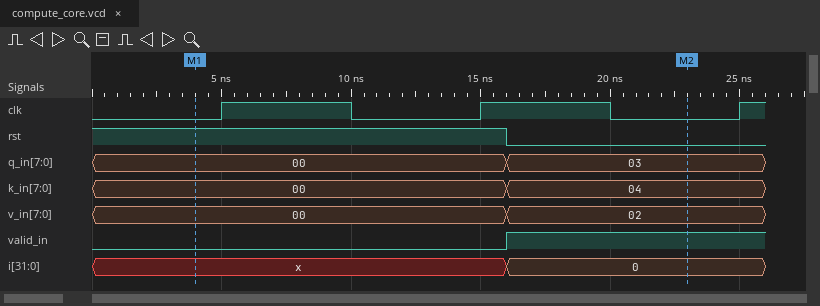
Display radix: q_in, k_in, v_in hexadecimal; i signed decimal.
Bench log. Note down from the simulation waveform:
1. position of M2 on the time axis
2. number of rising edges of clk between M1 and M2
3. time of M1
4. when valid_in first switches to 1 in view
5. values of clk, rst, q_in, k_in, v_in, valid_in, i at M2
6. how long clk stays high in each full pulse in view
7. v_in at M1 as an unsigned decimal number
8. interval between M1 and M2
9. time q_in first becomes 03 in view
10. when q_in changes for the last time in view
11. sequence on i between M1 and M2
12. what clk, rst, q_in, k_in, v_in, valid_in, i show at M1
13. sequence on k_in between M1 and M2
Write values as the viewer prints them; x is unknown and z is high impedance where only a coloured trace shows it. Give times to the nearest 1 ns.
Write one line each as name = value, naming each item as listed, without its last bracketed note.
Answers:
position of M2 on the time axis = 23 ns
number of rising edges of clk between M1 and M2 = 2
time of M1 = 4 ns
when valid_in first switches to 1 in view = 16 ns
values of clk, rst, q_in, k_in, v_in, valid_in, i at M2 = clk=0, rst=0, q_in=03, k_in=04, v_in=02, valid_in=1, i=0
how long clk stays high in each full pulse in view = 5 ns, 5 ns
v_in at M1 as an unsigned decimal number = 0
interval between M1 and M2 = 19 ns
time q_in first becomes 03 in view = 16 ns
when q_in changes for the last time in view = 16 ns
sequence on i between M1 and M2 = x, 0
what clk, rst, q_in, k_in, v_in, valid_in, i show at M1 = clk=0, rst=1, q_in=00, k_in=00, v_in=00, valid_in=0, i=x
sequence on k_in between M1 and M2 = 00, 04
